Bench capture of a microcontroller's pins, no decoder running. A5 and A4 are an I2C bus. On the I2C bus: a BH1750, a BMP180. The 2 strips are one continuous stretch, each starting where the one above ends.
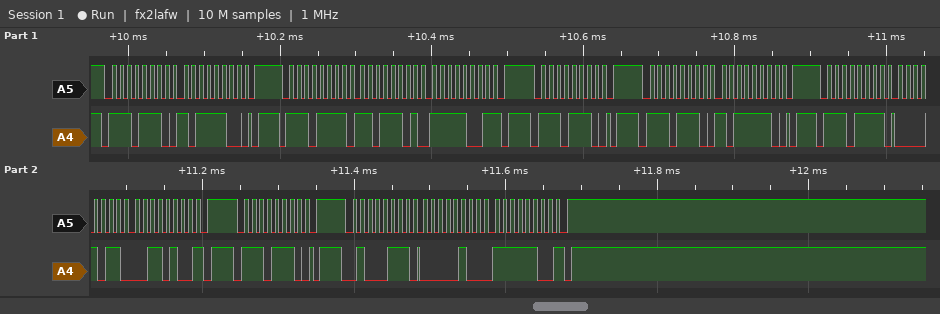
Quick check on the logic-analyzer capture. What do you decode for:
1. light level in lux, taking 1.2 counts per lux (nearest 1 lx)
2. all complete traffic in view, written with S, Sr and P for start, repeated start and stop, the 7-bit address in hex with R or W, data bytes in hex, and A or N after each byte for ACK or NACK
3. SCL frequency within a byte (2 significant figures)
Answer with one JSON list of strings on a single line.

["1063 lx", "S 77W A BC A P S 77R A DD A F9 N P S 77W A P S 77W A BE A P S 77R A 0B A 34 N P S 77W A P S 23R A 04 A FC N P", "100 kHz"]
